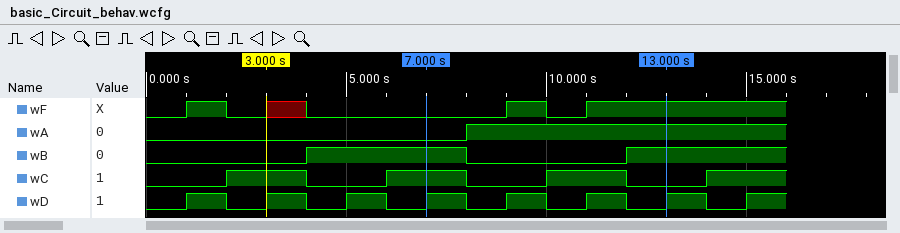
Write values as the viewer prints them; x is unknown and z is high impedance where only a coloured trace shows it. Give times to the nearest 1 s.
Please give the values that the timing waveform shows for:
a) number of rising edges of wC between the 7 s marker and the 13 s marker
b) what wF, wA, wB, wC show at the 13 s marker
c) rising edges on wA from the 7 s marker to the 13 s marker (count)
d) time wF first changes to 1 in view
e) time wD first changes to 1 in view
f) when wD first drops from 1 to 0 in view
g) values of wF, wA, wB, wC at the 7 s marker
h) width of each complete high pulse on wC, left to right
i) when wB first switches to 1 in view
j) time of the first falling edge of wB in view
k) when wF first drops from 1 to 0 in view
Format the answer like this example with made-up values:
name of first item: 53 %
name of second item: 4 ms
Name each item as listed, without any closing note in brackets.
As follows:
number of rising edges of wC between the 7 s marker and the 13 s marker: 1
what wF, wA, wB, wC show at the 13 s marker: wF=1, wA=1, wB=1, wC=0
rising edges on wA from the 7 s marker to the 13 s marker: 1
time wF first changes to 1 in view: 1 s
time wD first changes to 1 in view: 1 s
when wD first drops from 1 to 0 in view: 2 s
values of wF, wA, wB, wC at the 7 s marker: wF=0, wA=0, wB=1, wC=1
width of each complete high pulse on wC, left to right: 2 s, 2 s, 2 s
when wB first switches to 1 in view: 4 s
time of the first falling edge of wB in view: 8 s
when wF first drops from 1 to 0 in view: 2 s
